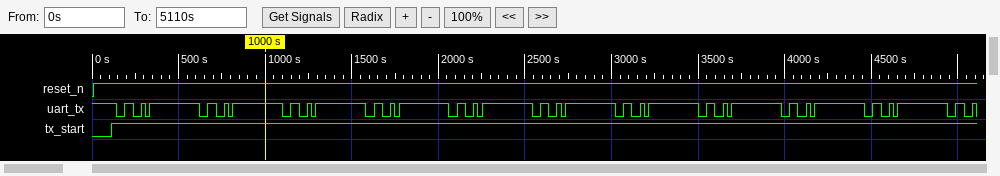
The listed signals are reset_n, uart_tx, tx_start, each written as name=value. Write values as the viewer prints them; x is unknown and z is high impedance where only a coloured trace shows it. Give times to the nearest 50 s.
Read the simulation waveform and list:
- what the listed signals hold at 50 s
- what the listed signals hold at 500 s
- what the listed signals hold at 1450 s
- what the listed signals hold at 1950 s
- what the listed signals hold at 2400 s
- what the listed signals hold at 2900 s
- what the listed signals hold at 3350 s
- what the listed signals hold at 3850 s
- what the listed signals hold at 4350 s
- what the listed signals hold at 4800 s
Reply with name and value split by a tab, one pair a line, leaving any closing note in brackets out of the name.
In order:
what the listed signals hold at 50 s	reset_n=1, uart_tx=1, tx_start=0
what the listed signals hold at 500 s	reset_n=1, uart_tx=1, tx_start=1
what the listed signals hold at 1450 s	reset_n=1, uart_tx=1, tx_start=1
what the listed signals hold at 1950 s	reset_n=1, uart_tx=1, tx_start=1
what the listed signals hold at 2400 s	reset_n=1, uart_tx=1, tx_start=1
what the listed signals hold at 2900 s	reset_n=1, uart_tx=1, tx_start=1
what the listed signals hold at 3350 s	reset_n=1, uart_tx=1, tx_start=1
what the listed signals hold at 3850 s	reset_n=1, uart_tx=1, tx_start=1
what the listed signals hold at 4350 s	reset_n=1, uart_tx=1, tx_start=1
what the listed signals hold at 4800 s	reset_n=1, uart_tx=1, tx_start=1
